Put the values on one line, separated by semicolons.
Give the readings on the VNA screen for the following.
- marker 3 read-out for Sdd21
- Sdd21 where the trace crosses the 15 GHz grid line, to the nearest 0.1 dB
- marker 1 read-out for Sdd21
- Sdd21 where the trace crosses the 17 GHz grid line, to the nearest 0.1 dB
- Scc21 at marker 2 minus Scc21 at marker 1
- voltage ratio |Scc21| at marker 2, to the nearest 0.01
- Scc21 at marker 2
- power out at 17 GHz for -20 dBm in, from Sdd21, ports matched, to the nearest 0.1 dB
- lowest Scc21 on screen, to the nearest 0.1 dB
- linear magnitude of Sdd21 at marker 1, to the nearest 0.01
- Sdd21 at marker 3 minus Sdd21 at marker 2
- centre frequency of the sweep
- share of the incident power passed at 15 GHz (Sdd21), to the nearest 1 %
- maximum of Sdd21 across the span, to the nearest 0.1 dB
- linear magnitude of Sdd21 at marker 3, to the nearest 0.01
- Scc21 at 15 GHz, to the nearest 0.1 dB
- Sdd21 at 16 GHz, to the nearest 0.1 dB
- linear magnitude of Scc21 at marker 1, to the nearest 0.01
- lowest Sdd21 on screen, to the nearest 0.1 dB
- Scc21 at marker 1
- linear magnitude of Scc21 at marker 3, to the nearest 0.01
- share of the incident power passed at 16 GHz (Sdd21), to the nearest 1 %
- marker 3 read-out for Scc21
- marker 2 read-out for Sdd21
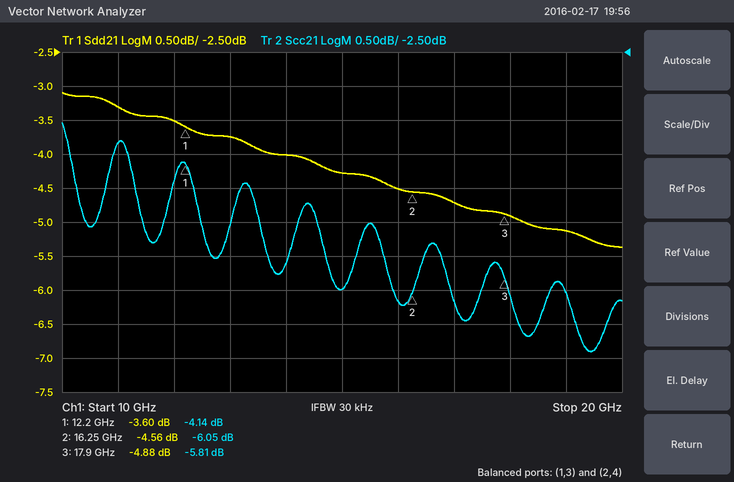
-4.88 dB; -4.3 dB; -3.60 dB; -4.7 dB; -1.91 dB; 0.50; -6.05 dB; -24.7 dBm; -6.9 dB; 0.66; -0.32 dB; 15 GHz; 37 %; -3.1 dB; 0.57; -6.0 dB; -4.5 dB; 0.62; -5.4 dB; -4.14 dB; 0.51; 35 %; -5.81 dB; -4.56 dB
